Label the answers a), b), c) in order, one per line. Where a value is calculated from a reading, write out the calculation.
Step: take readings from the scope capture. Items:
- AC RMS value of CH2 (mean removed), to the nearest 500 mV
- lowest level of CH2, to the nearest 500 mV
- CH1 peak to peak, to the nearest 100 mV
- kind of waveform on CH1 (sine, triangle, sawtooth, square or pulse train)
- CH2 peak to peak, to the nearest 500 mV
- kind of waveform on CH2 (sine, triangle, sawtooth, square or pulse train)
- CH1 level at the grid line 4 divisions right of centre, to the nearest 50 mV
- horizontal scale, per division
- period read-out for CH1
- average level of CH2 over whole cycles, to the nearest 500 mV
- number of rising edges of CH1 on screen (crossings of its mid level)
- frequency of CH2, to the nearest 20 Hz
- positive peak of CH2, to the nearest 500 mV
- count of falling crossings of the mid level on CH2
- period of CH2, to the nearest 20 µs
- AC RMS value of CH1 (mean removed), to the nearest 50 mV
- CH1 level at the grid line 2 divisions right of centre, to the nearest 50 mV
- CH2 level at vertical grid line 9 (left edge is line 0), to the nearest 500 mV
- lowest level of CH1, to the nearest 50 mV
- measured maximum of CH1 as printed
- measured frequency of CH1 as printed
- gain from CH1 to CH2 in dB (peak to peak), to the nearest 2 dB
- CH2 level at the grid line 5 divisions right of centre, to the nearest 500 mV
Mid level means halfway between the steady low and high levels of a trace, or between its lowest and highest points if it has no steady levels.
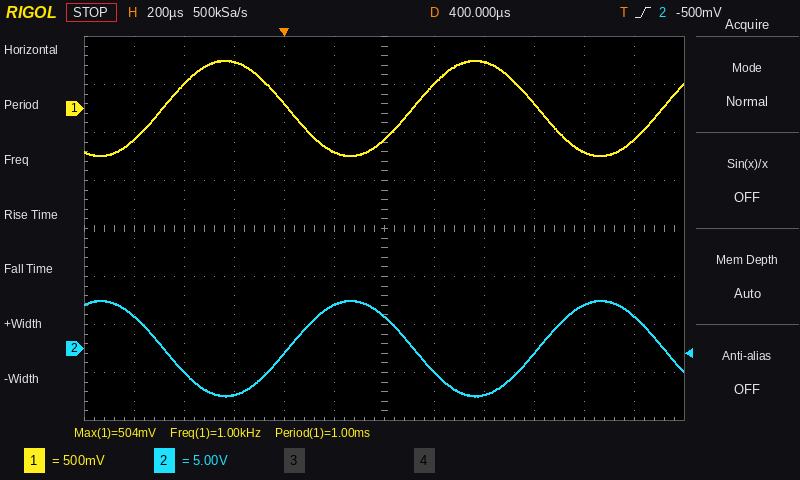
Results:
a) 10.0 V / (2√2) ≈ 3.5 V
b) -5.0 V
c) 1.00 V
d) sine
e) 5.0 V − (-5.0 V) = 10.0 V
f) sine
g) -450 mV
h) 200 µs
i) 1.00 ms
j) (5.0 V + (-5.0 V)) / 2 ≈ 0.0 V
k) 3
l) 1 / 1.00 ms ≈ 1.00 kHz
m) 5.0 V
n) 3
o) 1.00 ms
p) 1.00 V / (2√2) ≈ 354 mV, so 350 mV to the nearest 50 mV
q) 500 mV
r) -500 mV
s) -500 mV
t) 504 mV
u) 1.00 kHz
v) 20 log10(10.0 V / 1.00 V) ≈ 20 dB
w) 3.5 V
